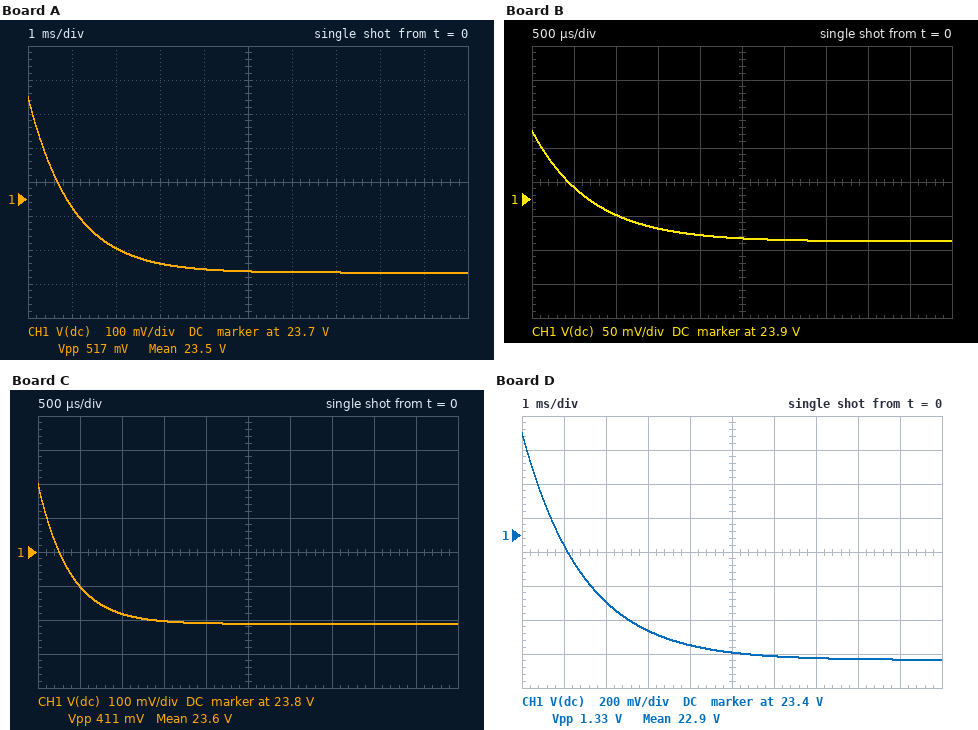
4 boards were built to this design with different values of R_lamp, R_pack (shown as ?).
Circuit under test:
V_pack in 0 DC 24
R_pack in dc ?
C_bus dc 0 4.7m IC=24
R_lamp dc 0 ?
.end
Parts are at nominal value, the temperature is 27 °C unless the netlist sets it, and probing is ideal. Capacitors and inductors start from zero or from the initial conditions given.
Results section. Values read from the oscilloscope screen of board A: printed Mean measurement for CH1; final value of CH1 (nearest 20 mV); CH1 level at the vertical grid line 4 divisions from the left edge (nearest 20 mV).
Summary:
23.5 V
23.48 V
23.50 V
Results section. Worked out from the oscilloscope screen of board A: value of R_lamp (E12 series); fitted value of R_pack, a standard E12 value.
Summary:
10 Ω
0.22 Ω
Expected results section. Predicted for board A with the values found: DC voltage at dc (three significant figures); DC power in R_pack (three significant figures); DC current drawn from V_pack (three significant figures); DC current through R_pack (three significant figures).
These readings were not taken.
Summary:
23.5 V
1.21 W
2.35 A
2.35 A
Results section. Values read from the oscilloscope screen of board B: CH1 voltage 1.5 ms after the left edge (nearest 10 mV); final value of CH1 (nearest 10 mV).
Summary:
23.86 V
23.84 V
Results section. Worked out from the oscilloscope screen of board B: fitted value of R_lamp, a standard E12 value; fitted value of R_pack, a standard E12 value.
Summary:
22 Ω
0.15 Ω
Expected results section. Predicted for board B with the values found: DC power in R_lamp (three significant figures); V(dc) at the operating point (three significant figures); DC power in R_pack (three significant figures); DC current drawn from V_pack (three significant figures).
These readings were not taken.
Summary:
25.8 W
23.8 V
176 mW
1.08 A
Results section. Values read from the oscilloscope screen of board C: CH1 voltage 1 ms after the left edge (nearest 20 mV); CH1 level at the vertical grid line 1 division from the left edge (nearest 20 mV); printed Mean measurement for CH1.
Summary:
23.62 V
23.70 V
23.6 V
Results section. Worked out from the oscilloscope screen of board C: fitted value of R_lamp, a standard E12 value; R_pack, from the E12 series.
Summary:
4.7 Ω
0.082 Ω
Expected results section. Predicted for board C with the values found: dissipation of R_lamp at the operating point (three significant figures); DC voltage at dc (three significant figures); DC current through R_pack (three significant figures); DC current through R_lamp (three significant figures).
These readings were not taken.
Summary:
118 W
23.6 V
5.02 A
5.02 A
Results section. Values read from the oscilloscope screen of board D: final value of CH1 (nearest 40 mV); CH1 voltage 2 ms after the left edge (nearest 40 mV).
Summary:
22.68 V
23.00 V
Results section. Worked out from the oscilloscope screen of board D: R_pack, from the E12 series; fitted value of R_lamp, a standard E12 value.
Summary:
0.33 Ω
5.6 Ω
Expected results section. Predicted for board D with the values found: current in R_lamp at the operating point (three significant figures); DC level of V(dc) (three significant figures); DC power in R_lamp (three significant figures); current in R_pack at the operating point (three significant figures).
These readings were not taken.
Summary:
4.05 A
22.7 V
91.7 W
4.05 A
